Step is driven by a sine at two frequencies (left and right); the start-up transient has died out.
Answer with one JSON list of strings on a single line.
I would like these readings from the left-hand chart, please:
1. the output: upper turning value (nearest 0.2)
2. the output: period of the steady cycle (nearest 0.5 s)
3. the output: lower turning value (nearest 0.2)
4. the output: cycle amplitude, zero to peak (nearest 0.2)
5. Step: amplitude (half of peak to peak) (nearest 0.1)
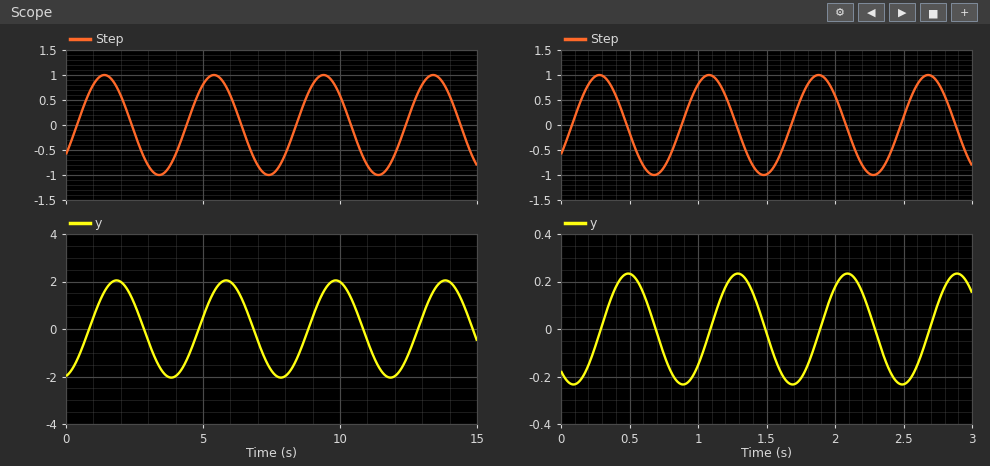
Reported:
["2.0", "4.0 s", "-2.0", "2.0", "1.0"]
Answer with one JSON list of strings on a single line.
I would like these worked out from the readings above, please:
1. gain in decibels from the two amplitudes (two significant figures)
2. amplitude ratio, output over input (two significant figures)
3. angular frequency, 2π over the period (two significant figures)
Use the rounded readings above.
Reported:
["6.0 dB", "2.0", "1.6 rad/s"]
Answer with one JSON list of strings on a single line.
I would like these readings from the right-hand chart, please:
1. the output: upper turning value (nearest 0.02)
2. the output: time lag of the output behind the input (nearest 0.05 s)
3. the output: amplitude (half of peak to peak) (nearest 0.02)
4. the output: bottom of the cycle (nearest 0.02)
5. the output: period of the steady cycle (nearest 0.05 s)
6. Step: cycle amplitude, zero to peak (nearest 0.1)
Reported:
["0.24", "0.20 s", "0.24", "-0.24", "0.80 s", "1.0"]
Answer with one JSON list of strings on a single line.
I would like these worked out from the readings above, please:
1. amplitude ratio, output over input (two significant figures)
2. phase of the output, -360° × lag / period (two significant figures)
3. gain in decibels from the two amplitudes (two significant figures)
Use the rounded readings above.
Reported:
["0.24", "-90°", "-12 dB"]
